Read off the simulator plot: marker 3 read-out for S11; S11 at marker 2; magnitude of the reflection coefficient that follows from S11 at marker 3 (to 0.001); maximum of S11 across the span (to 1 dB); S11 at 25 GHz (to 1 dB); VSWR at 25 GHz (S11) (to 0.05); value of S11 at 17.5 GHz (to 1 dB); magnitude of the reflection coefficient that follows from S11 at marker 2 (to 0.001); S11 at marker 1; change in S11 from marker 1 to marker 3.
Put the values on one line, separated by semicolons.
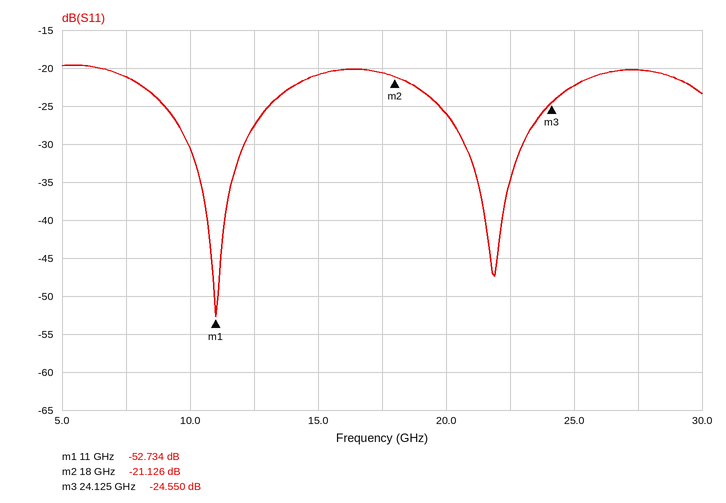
-24.550 dB; -21.126 dB; 0.059; -20 dB; -22 dB; 1.15; -21 dB; 0.088; -52.734 dB; 28.184 dB
